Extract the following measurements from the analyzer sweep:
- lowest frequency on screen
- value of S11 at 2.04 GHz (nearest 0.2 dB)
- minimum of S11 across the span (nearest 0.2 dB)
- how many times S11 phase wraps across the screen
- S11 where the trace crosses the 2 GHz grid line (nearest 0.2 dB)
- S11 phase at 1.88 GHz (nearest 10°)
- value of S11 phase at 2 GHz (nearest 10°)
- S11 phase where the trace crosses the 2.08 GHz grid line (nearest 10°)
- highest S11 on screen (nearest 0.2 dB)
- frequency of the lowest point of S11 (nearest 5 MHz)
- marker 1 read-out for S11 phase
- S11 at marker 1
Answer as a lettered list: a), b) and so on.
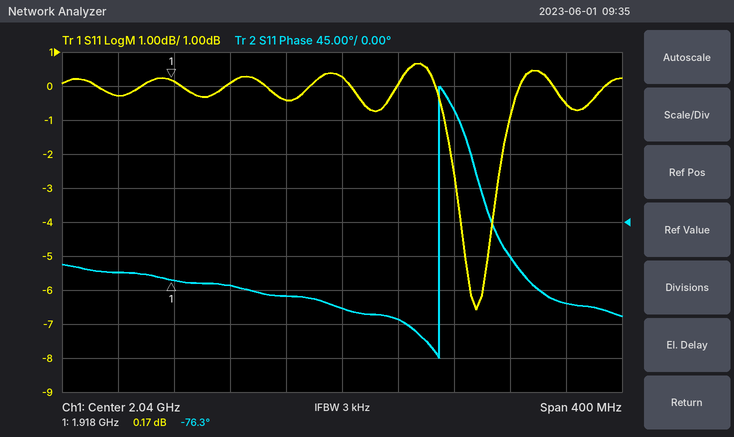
a) 1.84 GHz
b) 0.2 dB
c) -6.6 dB
d) 1
e) -0.4 dB
f) -70°
g) -100°
h) -130°
i) 0.6 dB
j) 2.135 GHz
k) -76.3°
l) 0.17 dB
